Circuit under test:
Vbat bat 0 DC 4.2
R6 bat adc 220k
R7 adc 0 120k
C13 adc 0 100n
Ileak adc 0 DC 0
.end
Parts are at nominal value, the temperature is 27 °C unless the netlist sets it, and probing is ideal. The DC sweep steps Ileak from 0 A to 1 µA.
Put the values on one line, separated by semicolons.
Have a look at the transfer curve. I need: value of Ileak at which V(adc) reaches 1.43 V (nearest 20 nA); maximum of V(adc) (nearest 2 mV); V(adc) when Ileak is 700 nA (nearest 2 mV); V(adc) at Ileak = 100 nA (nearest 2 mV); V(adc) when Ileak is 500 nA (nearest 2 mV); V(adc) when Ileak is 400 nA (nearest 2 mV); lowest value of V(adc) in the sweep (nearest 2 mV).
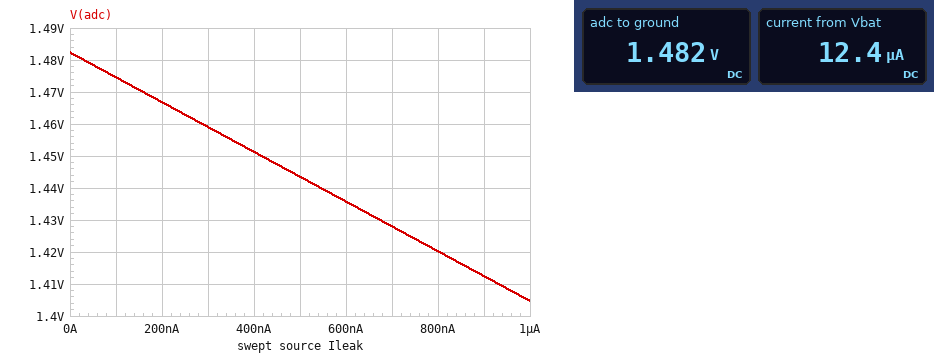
680 nA; 1.482 V; 1.428 V; 1.474 V; 1.444 V; 1.452 V; 1.404 V
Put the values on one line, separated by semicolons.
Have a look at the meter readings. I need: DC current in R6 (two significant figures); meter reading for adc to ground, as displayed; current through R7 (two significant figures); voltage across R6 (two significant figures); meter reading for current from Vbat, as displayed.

12 µA; 1.482 V; 12 µA; 2.7 V; 12.4 µA
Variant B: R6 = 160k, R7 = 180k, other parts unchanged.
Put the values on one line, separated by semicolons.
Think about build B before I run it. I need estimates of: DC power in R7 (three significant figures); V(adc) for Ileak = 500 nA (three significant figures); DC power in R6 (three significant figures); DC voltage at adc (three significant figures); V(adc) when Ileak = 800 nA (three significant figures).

27.5 µW; 2.18 V; 24.4 µW; 2.22 V; 2.16 V
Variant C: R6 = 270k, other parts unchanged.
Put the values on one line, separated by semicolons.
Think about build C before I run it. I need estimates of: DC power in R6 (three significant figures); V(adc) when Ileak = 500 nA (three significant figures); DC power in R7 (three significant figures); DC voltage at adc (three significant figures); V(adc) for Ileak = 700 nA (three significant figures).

31.3 µW; 1.25 V; 13.9 µW; 1.29 V; 1.23 V
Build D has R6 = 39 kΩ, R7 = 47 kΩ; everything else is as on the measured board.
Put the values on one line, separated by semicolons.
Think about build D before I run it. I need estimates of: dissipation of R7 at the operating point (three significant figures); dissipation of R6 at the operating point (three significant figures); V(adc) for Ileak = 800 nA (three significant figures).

112 µW; 93.0 µW; 2.28 V
